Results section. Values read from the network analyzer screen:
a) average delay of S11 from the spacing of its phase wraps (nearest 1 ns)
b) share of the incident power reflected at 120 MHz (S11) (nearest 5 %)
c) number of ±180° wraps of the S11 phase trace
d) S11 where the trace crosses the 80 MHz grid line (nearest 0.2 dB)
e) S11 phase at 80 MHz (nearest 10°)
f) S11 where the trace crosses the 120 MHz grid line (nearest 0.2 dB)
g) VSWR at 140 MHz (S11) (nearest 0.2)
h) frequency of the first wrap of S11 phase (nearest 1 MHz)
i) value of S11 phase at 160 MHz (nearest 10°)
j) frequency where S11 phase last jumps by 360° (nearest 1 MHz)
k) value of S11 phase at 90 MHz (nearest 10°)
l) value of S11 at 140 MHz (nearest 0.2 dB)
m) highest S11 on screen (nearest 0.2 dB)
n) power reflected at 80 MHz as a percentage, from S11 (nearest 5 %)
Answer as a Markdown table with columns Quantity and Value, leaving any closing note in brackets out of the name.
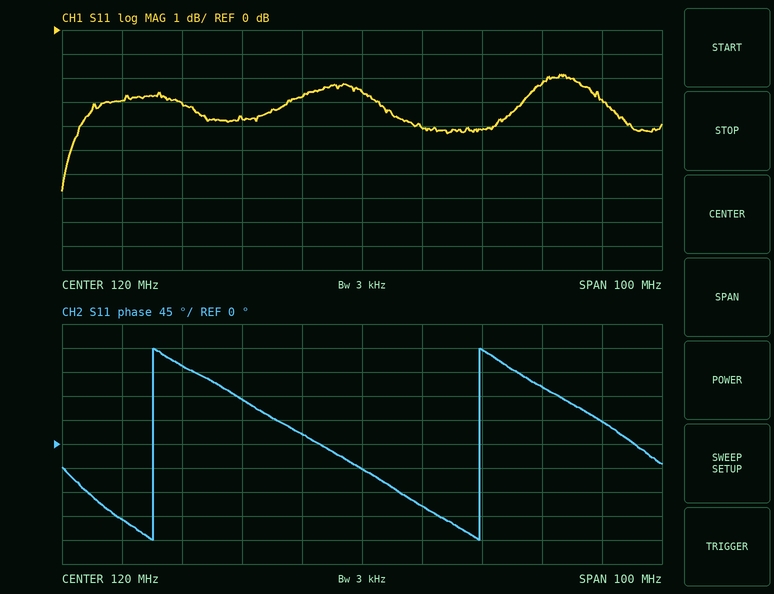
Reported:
| Quantity | Value |
|---|---|
| average delay of S11 from the spacing of its phase wraps | 18 ns |
| share of the incident power reflected at 120 MHz (S11) | 55 % |
| number of ±180° wraps of the S11 phase trace | 2 |
| S11 where the trace crosses the 80 MHz grid line | -3.0 dB |
| S11 phase at 80 MHz | -140° |
| S11 where the trace crosses the 120 MHz grid line | -2.6 dB |
| VSWR at 140 MHz (S11) | 4.2 |
| frequency of the first wrap of S11 phase | 85 MHz |
| value of S11 phase at 160 MHz | 40° |
| frequency where S11 phase last jumps by 360° | 140 MHz |
| value of S11 phase at 90 MHz | 150° |
| value of S11 at 140 MHz | -4.2 dB |
| highest S11 on screen | -1.8 dB |
| power reflected at 80 MHz as a percentage, from S11 | 50 % |
